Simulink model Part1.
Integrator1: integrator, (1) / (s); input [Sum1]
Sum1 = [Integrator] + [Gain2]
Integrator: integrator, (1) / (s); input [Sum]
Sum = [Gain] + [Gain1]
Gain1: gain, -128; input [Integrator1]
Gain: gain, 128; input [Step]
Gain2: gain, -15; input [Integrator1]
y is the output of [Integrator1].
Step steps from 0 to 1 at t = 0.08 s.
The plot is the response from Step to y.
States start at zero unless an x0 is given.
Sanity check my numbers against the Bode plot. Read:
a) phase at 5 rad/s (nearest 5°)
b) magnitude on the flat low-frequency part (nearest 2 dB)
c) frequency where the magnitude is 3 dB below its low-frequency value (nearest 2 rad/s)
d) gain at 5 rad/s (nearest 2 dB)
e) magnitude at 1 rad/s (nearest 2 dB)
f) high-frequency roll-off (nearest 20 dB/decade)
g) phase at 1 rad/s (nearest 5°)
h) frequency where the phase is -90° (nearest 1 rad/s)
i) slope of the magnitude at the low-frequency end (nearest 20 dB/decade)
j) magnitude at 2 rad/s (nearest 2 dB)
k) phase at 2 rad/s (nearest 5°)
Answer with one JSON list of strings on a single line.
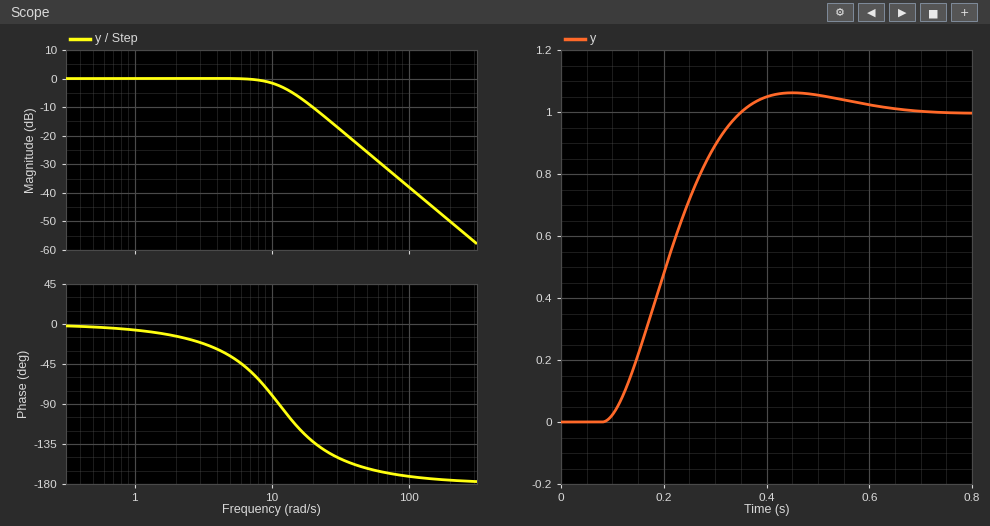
["-35°", "0 dB", "12 rad/s", "0 dB", "0 dB", "-40 dB/decade", "-5°", "11 rad/s", "0 dB/decade", "0 dB", "-15°"]
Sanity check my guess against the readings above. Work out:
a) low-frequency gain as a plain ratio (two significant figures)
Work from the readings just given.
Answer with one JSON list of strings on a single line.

["1.0"]
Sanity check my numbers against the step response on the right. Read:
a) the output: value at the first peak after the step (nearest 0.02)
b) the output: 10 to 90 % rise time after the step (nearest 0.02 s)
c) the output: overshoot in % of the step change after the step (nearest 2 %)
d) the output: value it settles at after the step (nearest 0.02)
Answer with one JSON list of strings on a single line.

["1.06", "0.18 s", "6 %", "1.00"]
